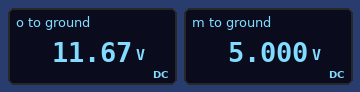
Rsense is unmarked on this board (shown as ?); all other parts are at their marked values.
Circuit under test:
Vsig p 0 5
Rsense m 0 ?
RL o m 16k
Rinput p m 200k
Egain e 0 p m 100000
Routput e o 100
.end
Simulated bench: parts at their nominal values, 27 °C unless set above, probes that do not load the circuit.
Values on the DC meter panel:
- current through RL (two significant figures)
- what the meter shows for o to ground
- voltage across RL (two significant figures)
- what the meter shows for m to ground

420 µA
11.67 V
6.7 V
5.000 V
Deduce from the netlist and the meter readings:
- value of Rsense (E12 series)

12 kΩ
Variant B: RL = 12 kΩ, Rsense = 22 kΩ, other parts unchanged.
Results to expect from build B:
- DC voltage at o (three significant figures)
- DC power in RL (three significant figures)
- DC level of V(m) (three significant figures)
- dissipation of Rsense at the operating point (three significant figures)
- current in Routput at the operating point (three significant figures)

7.73 V
620 µW
5.00 V
1.14 mW
227 µA
